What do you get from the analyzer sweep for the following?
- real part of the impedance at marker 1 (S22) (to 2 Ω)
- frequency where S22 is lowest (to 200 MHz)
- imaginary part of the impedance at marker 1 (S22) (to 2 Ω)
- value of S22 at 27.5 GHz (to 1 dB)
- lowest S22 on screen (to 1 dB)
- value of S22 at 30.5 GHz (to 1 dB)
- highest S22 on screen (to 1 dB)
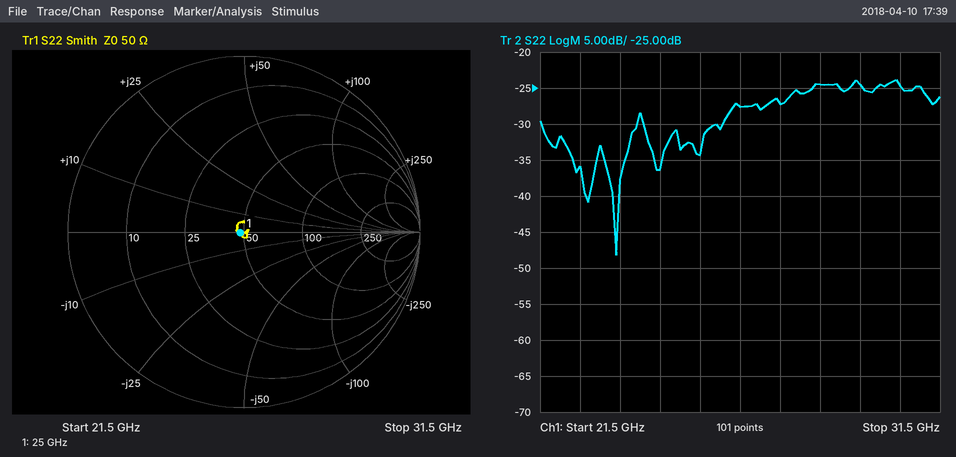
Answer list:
48 Ω
23.4 GHz
0 Ω
-27 dB
-48 dB
-25 dB
-24 dB
